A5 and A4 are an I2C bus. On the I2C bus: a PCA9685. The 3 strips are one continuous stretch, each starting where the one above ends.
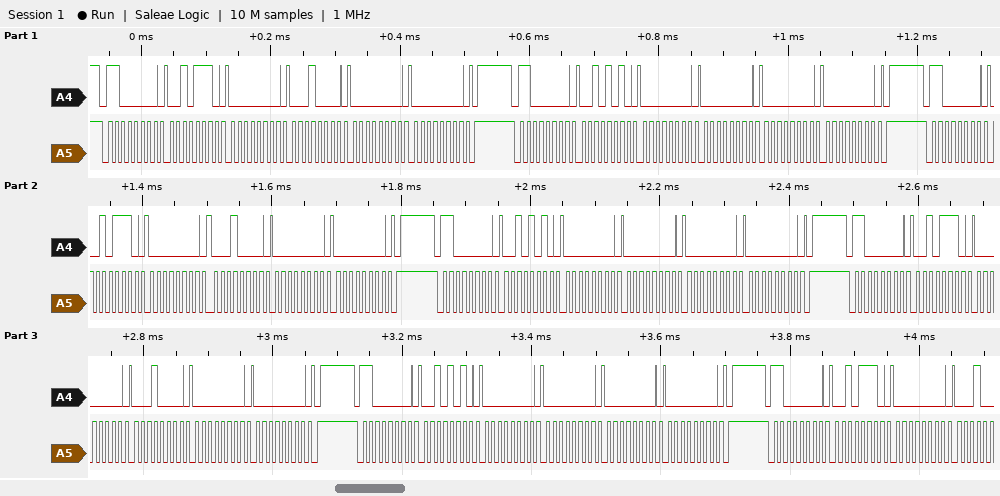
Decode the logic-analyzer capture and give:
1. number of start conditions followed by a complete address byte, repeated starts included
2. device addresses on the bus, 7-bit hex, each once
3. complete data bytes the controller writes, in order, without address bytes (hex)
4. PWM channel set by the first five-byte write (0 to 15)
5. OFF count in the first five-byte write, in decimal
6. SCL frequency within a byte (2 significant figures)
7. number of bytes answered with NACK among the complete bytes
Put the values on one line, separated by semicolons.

7; 0x60; 2E 00 10 00 00 2A 00 00 00 00 2E 00 10 00 00 2A 00 00 00 00 2E 00 10 00 00 2A 00 00 00 00 2E 00; 10; 0; 100 kHz; 0
